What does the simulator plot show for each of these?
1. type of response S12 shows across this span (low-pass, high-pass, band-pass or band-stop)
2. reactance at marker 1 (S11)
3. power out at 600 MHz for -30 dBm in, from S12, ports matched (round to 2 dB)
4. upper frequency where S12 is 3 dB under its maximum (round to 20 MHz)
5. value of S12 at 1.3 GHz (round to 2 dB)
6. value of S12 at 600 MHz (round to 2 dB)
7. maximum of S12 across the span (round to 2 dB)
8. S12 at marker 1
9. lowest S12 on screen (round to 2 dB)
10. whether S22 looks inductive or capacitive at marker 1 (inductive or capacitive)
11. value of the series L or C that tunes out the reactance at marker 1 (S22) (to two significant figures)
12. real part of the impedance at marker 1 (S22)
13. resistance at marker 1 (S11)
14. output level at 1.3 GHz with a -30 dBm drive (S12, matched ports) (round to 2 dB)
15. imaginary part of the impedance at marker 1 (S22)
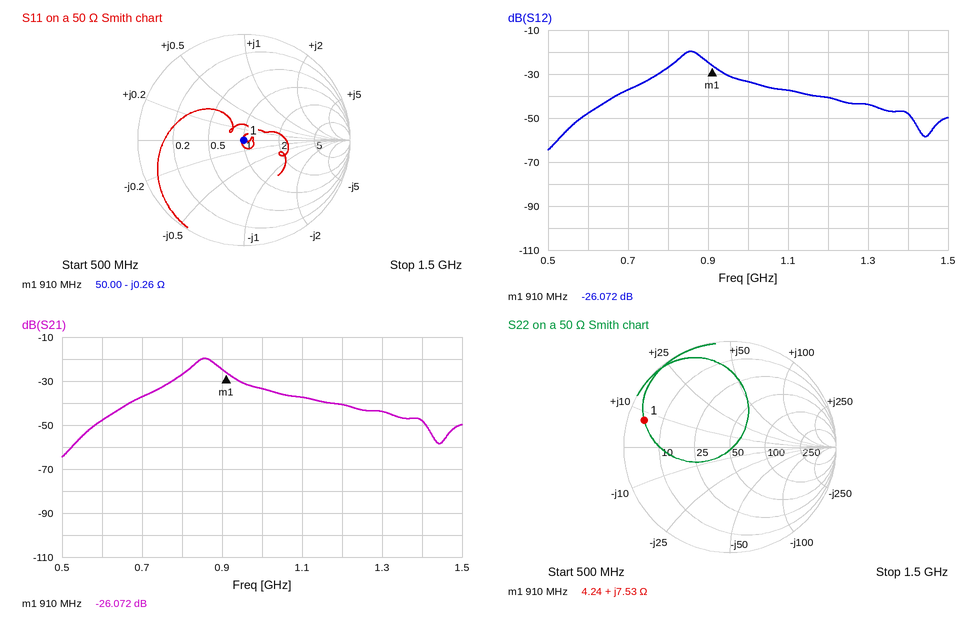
band-pass
-0.26 Ω
-78 dBm
880 MHz
-44 dB
-48 dB
-20 dB
-26.072 dB
-64 dB
inductive
23 pF
4.24 Ω
50.00 Ω
-74 dBm
+7.53 Ω
